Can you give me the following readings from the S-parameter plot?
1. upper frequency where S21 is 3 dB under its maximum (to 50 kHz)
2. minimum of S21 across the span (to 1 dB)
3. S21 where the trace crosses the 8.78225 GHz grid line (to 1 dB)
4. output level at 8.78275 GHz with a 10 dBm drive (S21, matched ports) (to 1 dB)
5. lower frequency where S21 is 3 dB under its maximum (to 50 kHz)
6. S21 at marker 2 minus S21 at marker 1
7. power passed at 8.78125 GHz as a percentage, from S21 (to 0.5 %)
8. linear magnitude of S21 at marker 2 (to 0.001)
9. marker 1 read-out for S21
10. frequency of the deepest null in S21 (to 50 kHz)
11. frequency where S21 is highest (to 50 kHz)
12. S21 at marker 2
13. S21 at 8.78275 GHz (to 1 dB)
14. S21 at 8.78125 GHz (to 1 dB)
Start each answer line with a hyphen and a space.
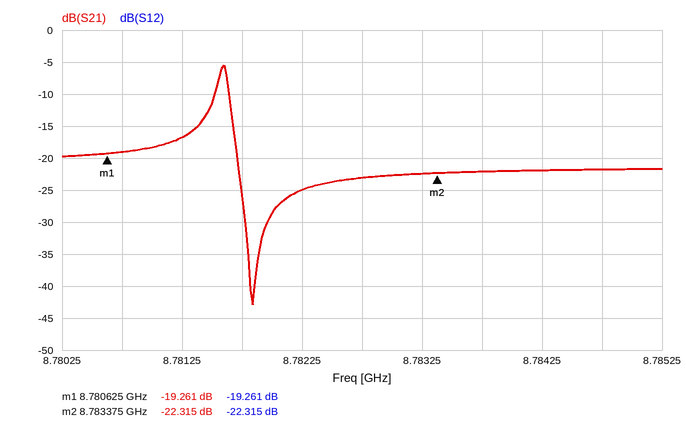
- 8.78165 GHz
- -43 dB
- -25 dB
- -13 dBm
- 8.78155 GHz
- -3.054 dB
- 2.0 %
- 0.077
- -19.261 dB
- 8.78185 GHz
- 8.78160 GHz
- -22.315 dB
- -23 dB
- -17 dB
